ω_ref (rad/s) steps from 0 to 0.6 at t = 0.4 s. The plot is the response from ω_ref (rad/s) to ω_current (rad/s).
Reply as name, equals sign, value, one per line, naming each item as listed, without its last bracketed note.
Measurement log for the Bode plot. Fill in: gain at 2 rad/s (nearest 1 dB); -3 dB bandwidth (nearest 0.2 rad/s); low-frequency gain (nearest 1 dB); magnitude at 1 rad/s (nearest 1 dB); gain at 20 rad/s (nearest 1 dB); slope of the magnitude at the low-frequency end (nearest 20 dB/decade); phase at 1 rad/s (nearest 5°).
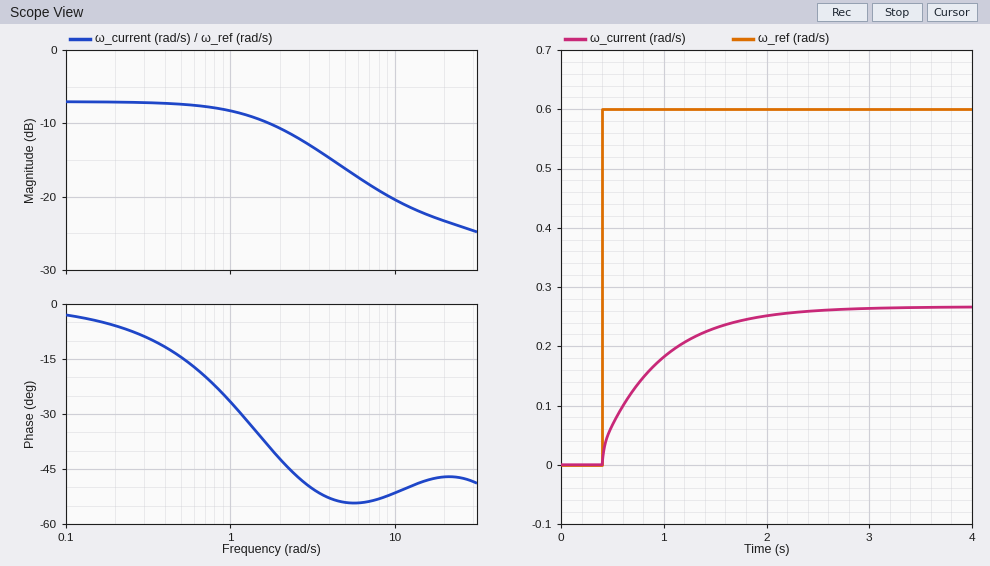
gain at 2 rad/s = -11 dB
-3 dB bandwidth = 1.8 rad/s
low-frequency gain = -7 dB
magnitude at 1 rad/s = -8 dB
gain at 20 rad/s = -23 dB
slope of the magnitude at the low-frequency end = 0 dB/decade
phase at 1 rad/s = -25°
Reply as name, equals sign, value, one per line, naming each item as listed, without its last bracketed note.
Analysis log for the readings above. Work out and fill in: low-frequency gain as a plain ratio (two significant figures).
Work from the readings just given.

low-frequency gain as a plain ratio = 0.45
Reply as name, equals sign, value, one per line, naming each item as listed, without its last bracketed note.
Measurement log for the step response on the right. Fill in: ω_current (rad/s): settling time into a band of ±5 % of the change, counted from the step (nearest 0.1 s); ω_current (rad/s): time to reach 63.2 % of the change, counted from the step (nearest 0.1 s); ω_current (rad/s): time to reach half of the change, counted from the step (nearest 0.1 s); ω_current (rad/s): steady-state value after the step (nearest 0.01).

ω_current (rad/s): settling time into a band of ±5 % of the change, counted from the step = 1.7 s
ω_current (rad/s): time to reach 63.2 % of the change, counted from the step = 0.5 s
ω_current (rad/s): time to reach half of the change, counted from the step = 0.3 s
ω_current (rad/s): steady-state value after the step = 0.27
